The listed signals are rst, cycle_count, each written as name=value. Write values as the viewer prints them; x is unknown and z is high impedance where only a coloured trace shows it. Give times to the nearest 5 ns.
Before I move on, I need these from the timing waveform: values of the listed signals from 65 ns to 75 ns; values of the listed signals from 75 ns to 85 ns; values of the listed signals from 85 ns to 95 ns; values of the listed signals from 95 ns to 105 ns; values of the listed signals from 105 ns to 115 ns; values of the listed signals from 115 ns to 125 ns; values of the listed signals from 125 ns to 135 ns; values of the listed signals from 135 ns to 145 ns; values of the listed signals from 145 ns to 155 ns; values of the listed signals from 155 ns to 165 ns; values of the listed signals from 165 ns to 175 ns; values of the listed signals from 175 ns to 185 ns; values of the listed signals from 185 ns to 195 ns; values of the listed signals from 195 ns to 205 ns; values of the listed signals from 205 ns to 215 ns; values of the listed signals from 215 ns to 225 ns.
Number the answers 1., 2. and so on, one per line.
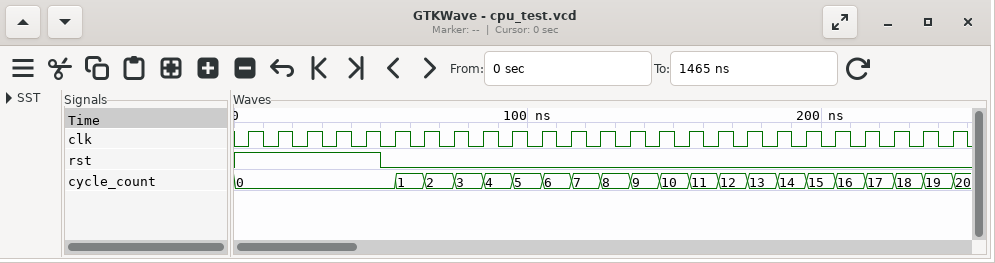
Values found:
1. rst=0, cycle_count=2
2. rst=0, cycle_count=3
3. rst=0, cycle_count=4
4. rst=0, cycle_count=5
5. rst=0, cycle_count=6
6. rst=0, cycle_count=7
7. rst=0, cycle_count=8
8. rst=0, cycle_count=9
9. rst=0, cycle_count=10
10. rst=0, cycle_count=11
11. rst=0, cycle_count=12
12. rst=0, cycle_count=13
13. rst=0, cycle_count=14
14. rst=0, cycle_count=15
15. rst=0, cycle_count=16
16. rst=0, cycle_count=17
